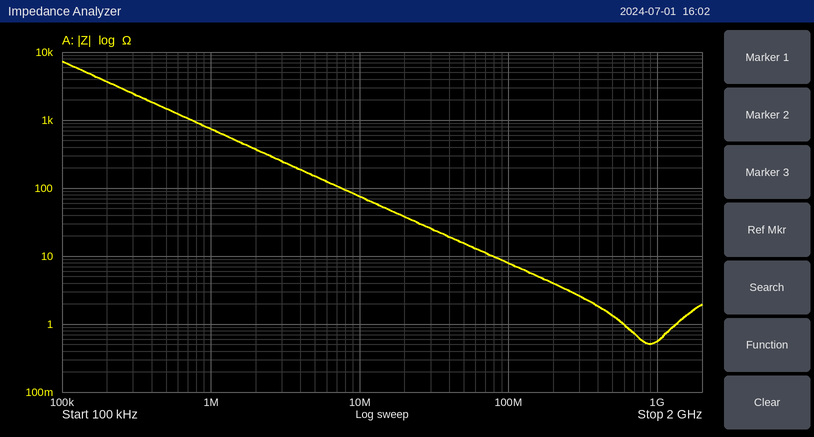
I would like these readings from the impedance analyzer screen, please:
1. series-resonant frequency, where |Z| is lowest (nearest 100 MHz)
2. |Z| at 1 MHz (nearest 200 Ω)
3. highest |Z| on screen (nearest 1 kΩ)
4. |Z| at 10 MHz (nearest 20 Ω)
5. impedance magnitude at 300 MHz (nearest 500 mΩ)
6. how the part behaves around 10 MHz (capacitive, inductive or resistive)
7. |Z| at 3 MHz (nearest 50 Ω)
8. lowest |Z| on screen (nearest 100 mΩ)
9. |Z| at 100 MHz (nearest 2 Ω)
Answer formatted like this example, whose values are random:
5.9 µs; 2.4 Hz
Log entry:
900 MHz; 800 Ω; 7 kΩ; 80 Ω; 2.5 Ω; capacitive; 250 Ω; 500 mΩ; 8 Ω
